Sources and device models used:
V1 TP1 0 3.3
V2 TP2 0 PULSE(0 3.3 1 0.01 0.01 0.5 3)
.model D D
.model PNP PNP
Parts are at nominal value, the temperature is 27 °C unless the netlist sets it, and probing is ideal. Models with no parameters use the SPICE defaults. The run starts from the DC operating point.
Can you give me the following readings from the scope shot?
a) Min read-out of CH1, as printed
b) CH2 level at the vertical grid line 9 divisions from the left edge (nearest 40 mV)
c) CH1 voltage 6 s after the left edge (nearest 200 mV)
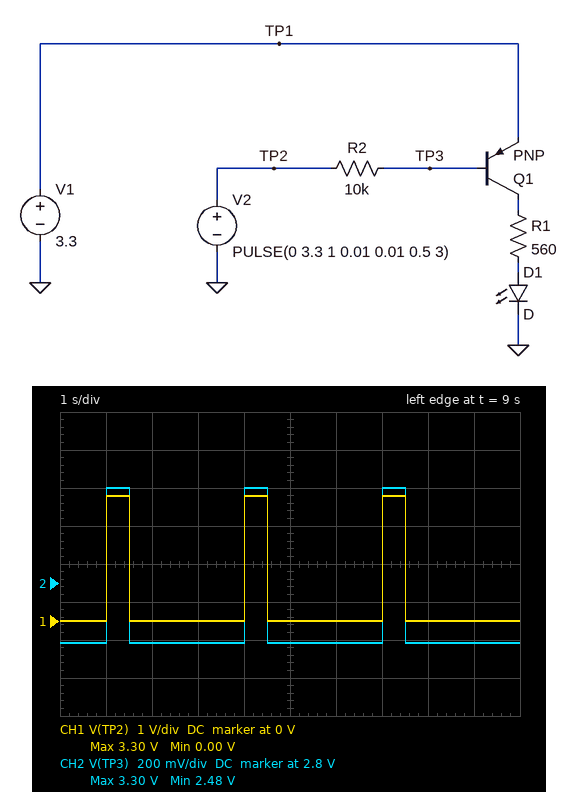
0.00 V
2.48 V
0 V
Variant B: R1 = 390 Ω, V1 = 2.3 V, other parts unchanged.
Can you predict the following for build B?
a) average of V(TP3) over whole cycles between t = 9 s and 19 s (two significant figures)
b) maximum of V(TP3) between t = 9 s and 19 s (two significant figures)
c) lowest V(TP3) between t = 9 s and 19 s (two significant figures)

1.8 V
3.3 V
1.5 V
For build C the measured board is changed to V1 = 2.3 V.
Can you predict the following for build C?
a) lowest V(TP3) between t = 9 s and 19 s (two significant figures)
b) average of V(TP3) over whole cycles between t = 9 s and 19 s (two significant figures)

1.5 V
1.8 V
